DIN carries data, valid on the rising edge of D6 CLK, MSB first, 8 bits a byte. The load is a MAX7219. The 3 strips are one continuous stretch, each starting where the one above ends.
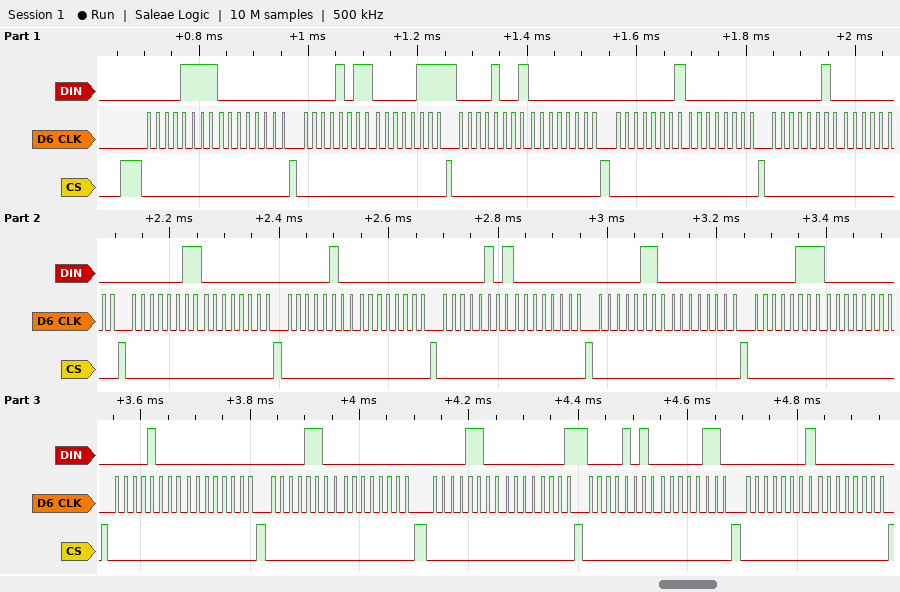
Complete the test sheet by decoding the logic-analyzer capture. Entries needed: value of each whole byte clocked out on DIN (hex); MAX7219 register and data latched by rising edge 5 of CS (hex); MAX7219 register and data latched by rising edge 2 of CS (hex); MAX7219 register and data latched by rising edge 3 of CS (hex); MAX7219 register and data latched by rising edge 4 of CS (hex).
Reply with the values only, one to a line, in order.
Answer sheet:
0F 00 0B 07 09 00 01 00 02 00 03 00 04 00 05 00 06 00 07 00 08 00 0C 00 0C 01 0A 06 01 00
register 0x1, data 0x00
register 0xF, data 0x00
register 0xB, data 0x07
register 0x9, data 0x00
